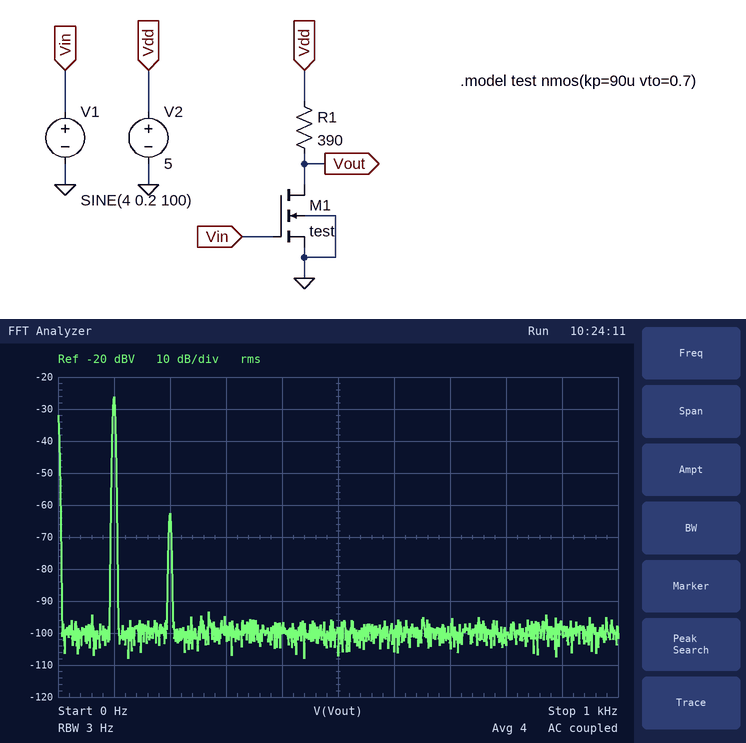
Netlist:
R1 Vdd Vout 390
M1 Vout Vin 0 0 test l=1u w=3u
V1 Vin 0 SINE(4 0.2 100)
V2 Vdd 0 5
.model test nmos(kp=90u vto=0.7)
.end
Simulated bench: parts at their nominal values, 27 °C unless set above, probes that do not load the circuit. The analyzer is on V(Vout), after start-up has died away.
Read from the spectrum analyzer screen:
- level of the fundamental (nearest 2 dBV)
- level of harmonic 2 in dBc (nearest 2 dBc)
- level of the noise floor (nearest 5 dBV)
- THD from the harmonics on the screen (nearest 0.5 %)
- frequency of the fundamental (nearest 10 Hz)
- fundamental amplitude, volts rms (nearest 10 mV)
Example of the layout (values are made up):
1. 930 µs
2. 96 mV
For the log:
1. -26 dBV
2. -36 dBc
3. -100 dBV
4. 1.5 %
5. 100 Hz
6. 50 mV
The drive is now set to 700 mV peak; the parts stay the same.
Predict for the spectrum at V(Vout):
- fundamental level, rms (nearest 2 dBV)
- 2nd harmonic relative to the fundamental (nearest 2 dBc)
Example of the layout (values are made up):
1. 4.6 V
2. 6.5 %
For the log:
1. -16 dBV
2. -26 dBc
